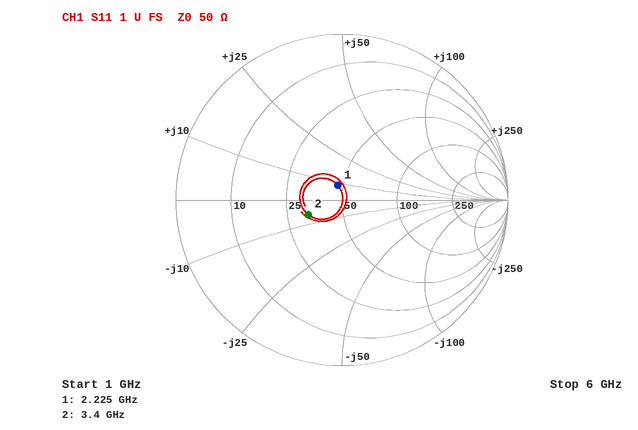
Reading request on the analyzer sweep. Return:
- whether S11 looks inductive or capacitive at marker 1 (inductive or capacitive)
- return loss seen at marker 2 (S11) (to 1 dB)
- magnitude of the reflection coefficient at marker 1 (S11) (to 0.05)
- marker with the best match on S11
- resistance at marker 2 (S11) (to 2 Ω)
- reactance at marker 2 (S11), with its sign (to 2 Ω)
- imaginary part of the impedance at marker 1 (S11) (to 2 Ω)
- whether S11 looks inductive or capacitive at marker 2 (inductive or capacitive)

inductive
13 dB
0.10
marker 1
32 Ω
-6 Ω
+8 Ω
capacitive
